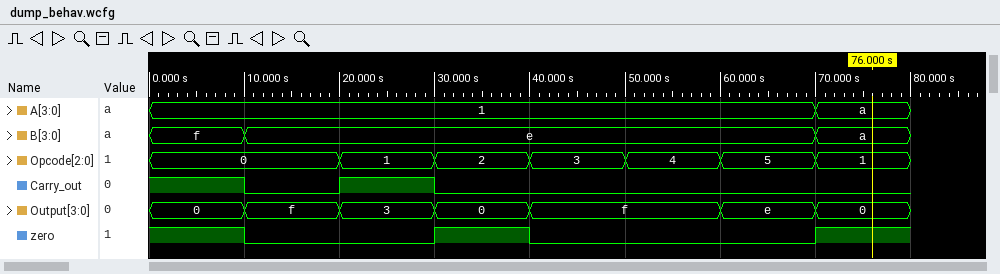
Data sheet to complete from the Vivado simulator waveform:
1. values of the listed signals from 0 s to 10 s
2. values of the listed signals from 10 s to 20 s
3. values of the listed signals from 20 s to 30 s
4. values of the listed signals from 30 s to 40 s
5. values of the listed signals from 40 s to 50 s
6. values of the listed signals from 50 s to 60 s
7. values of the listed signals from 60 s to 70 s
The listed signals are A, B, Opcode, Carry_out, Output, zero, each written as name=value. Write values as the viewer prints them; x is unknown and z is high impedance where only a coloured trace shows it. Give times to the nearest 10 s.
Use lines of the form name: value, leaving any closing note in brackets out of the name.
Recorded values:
values of the listed signals from 0 s to 10 s: A=1, B=f, Opcode=0, Carry_out=1, Output=0, zero=1
values of the listed signals from 10 s to 20 s: A=1, B=e, Opcode=0, Carry_out=0, Output=f, zero=0
values of the listed signals from 20 s to 30 s: A=1, B=e, Opcode=1, Carry_out=1, Output=3, zero=0
values of the listed signals from 30 s to 40 s: A=1, B=e, Opcode=2, Carry_out=0, Output=0, zero=1
values of the listed signals from 40 s to 50 s: A=1, B=e, Opcode=3, Carry_out=0, Output=f, zero=0
values of the listed signals from 50 s to 60 s: A=1, B=e, Opcode=4, Carry_out=0, Output=f, zero=0
values of the listed signals from 60 s to 70 s: A=1, B=e, Opcode=5, Carry_out=0, Output=e, zero=0
